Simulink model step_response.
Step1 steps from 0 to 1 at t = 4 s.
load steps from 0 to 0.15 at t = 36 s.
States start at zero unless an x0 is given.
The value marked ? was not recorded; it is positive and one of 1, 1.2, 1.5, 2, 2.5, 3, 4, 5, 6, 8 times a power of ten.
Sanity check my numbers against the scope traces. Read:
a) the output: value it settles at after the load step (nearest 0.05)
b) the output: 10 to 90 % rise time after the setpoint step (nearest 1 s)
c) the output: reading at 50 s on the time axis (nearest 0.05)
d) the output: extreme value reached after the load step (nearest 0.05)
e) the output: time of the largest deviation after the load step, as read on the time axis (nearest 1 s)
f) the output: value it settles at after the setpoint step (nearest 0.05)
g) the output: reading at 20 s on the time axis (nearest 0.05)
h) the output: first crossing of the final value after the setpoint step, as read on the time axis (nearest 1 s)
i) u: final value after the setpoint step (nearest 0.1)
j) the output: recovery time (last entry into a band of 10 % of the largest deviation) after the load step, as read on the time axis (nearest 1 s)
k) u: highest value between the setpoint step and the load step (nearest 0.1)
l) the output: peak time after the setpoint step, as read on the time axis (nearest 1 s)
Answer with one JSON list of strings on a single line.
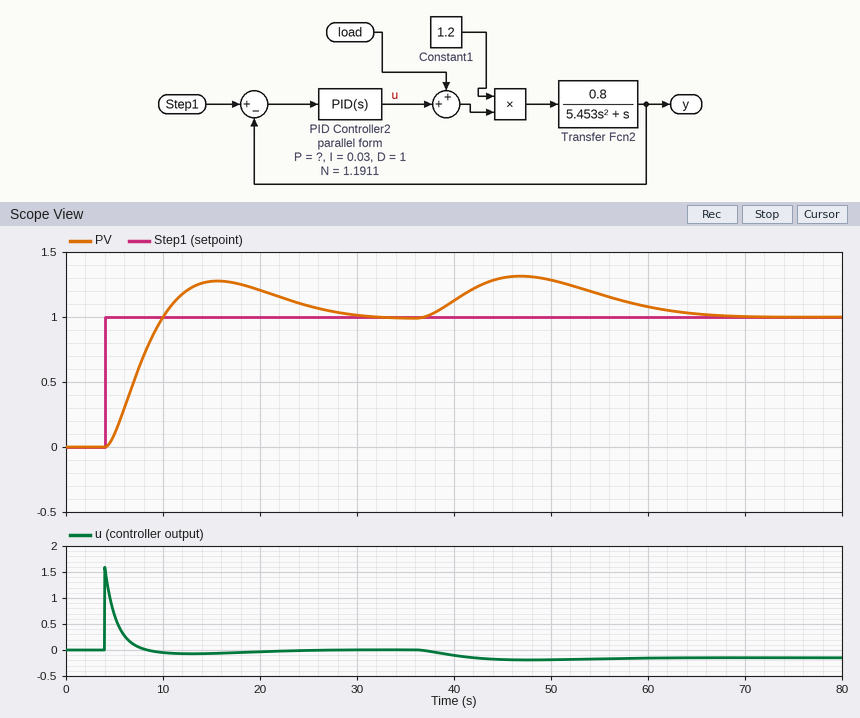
["1.00", "4 s", "1.30", "1.30", "47 s", "1.00", "1.20", "10 s", "0.0", "64 s", "1.6", "16 s"]
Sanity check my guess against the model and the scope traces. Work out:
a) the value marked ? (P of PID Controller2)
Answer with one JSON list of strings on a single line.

["0.4"]
